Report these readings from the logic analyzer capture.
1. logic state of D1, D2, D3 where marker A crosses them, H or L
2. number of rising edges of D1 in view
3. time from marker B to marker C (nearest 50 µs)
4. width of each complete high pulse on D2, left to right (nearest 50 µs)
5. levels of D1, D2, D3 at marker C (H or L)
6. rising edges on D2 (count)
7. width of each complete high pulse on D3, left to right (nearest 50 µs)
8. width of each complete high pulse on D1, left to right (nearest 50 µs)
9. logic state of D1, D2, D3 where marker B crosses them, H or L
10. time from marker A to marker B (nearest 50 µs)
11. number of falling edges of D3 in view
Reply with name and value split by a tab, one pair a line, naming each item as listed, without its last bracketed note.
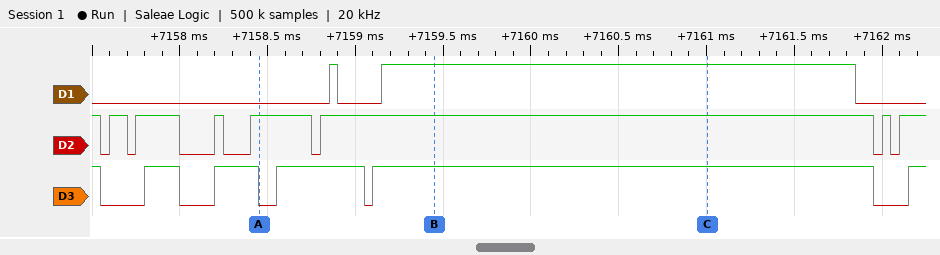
logic state of D1, D2, D3 where marker A crosses them, H or L	D1=L, D2=H, D3=L
number of rising edges of D1 in view	2
time from marker B to marker C	1550 µs
width of each complete high pulse on D2, left to right	100 µs, 250 µs, 50 µs, 350 µs, 3150 µs, 50 µs
levels of D1, D2, D3 at marker C	D1=H, D2=H, D3=H
rising edges on D2	7
width of each complete high pulse on D3, left to right	200 µs, 250 µs, 500 µs, 2850 µs
width of each complete high pulse on D1, left to right	50 µs, 2700 µs
logic state of D1, D2, D3 where marker B crosses them, H or L	D1=H, D2=H, D3=H
time from marker A to marker B	1000 µs
number of falling edges of D3 in view	5
